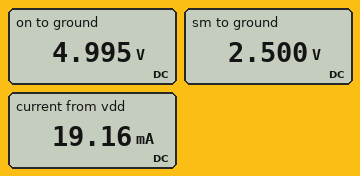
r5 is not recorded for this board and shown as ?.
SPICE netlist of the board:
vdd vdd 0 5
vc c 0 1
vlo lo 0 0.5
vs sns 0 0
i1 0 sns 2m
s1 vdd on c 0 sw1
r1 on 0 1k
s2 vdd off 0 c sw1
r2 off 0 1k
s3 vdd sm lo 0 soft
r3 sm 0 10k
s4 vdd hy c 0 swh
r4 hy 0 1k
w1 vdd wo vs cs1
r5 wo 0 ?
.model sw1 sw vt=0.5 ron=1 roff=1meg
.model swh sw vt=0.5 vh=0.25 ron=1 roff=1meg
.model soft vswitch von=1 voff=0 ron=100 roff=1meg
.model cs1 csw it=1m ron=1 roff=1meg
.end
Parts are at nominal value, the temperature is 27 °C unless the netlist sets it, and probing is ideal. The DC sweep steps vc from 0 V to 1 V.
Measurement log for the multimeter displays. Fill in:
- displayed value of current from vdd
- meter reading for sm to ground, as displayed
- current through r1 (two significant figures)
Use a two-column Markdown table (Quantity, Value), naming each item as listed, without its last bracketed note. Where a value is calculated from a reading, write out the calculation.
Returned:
| Quantity | Value |
|---|---|
| displayed value of current from vdd | 19.16 mA |
| meter reading for sm to ground, as displayed | 2.500 V |
| current through r1 | (4.995 V) / 1 kΩ = 5.0 mA |
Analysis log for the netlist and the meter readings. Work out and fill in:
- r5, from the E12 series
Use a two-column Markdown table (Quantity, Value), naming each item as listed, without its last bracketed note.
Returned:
| Quantity | Value |
|---|---|
| r5, from the E12 series | 560 Ω |
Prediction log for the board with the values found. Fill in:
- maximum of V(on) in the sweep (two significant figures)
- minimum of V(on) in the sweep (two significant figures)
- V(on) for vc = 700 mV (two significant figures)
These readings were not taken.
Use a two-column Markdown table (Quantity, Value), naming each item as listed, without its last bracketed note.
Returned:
| Quantity | Value |
|---|---|
| maximum of V(on) in the sweep | 5.0 V |
| minimum of V(on) in the sweep | 5.0 mV |
| V(on) for vc = 700 mV | 5.0 V |
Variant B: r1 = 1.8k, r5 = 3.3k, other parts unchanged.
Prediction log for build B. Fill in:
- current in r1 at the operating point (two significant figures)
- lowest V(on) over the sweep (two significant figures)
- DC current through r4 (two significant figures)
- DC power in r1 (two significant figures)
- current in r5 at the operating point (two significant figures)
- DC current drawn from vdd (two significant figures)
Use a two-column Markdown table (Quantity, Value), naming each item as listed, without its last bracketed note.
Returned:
| Quantity | Value |
|---|---|
| current in r1 at the operating point | 2.8 mA |
| lowest V(on) over the sweep | 9.0 mV |
| DC current through r4 | 5.0 mA |
| DC power in r1 | 14 mW |
| current in r5 at the operating point | 1.5 mA |
| DC current drawn from vdd | 9.5 mA |
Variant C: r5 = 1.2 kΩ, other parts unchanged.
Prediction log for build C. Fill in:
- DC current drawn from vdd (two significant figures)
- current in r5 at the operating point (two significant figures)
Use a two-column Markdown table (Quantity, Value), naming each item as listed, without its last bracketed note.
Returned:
| Quantity | Value |
|---|---|
| DC current drawn from vdd | 14 mA |
| current in r5 at the operating point | 4.2 mA |
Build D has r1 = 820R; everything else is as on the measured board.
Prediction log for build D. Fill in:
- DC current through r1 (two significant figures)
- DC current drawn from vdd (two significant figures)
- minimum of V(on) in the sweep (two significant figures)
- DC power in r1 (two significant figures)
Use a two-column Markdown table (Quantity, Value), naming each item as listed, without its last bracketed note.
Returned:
| Quantity | Value |
|---|---|
| DC current through r1 | 6.1 mA |
| DC current drawn from vdd | 20 mA |
| minimum of V(on) in the sweep | 4.1 mV |
| DC power in r1 | 30 mW |
